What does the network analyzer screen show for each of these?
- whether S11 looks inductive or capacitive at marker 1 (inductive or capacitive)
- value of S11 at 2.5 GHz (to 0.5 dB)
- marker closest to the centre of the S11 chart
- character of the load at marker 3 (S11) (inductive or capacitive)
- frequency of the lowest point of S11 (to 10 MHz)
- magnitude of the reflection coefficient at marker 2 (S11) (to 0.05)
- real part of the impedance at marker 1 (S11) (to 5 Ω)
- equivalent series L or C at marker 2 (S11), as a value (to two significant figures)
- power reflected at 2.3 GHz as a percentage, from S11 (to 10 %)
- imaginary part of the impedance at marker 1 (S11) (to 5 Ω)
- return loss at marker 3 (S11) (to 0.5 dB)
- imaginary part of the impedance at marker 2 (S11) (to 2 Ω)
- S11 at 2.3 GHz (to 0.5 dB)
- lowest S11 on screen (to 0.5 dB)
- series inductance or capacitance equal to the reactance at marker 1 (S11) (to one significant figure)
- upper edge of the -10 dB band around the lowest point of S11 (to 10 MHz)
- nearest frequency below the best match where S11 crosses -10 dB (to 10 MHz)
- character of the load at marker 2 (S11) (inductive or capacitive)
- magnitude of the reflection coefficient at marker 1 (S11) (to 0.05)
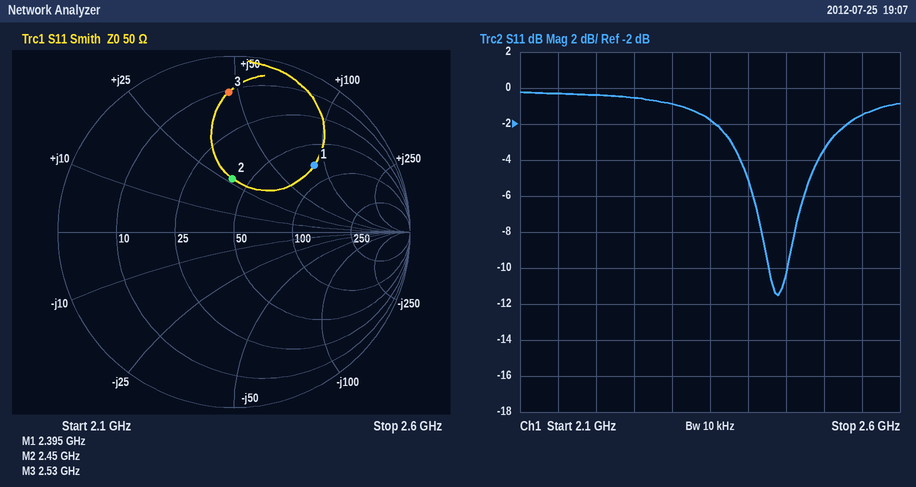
inductive
-3.5 dB
marker 2
inductive
2.44 GHz
0.30
75 Ω
1.8 nH
80 %
+85 Ω
2.0 dB
+28 Ω
-1.0 dB
-11.5 dB
6 nH
2.45 GHz
2.43 GHz
inductive
0.60
